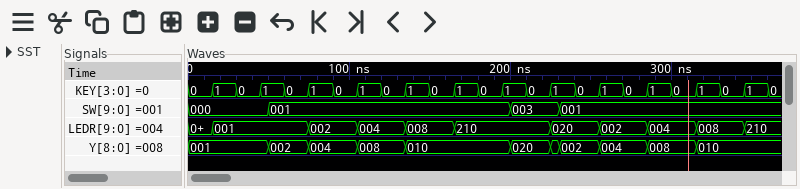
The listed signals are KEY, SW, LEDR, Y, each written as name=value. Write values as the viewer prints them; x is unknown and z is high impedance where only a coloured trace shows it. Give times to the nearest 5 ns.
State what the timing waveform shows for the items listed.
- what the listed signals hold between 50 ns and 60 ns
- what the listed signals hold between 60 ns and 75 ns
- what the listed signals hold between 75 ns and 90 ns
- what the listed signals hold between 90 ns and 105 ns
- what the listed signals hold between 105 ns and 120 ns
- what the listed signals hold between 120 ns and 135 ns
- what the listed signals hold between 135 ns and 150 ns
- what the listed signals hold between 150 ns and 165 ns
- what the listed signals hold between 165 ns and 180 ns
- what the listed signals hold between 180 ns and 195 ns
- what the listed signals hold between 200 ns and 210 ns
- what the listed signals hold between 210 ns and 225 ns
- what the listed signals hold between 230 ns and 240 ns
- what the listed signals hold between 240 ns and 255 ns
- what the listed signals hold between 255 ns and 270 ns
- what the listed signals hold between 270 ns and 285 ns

KEY=1, SW=001, LEDR=001, Y=002
KEY=0, SW=001, LEDR=001, Y=002
KEY=1, SW=001, LEDR=002, Y=004
KEY=0, SW=001, LEDR=002, Y=004
KEY=1, SW=001, LEDR=004, Y=008
KEY=0, SW=001, LEDR=004, Y=008
KEY=1, SW=001, LEDR=008, Y=010
KEY=0, SW=001, LEDR=008, Y=010
KEY=1, SW=001, LEDR=210, Y=010
KEY=0, SW=001, LEDR=210, Y=010
KEY=1, SW=003, LEDR=210, Y=020
KEY=0, SW=003, LEDR=210, Y=020
KEY=1, SW=001, LEDR=020, Y=002
KEY=0, SW=001, LEDR=020, Y=002
KEY=1, SW=001, LEDR=002, Y=004
KEY=0, SW=001, LEDR=002, Y=004
